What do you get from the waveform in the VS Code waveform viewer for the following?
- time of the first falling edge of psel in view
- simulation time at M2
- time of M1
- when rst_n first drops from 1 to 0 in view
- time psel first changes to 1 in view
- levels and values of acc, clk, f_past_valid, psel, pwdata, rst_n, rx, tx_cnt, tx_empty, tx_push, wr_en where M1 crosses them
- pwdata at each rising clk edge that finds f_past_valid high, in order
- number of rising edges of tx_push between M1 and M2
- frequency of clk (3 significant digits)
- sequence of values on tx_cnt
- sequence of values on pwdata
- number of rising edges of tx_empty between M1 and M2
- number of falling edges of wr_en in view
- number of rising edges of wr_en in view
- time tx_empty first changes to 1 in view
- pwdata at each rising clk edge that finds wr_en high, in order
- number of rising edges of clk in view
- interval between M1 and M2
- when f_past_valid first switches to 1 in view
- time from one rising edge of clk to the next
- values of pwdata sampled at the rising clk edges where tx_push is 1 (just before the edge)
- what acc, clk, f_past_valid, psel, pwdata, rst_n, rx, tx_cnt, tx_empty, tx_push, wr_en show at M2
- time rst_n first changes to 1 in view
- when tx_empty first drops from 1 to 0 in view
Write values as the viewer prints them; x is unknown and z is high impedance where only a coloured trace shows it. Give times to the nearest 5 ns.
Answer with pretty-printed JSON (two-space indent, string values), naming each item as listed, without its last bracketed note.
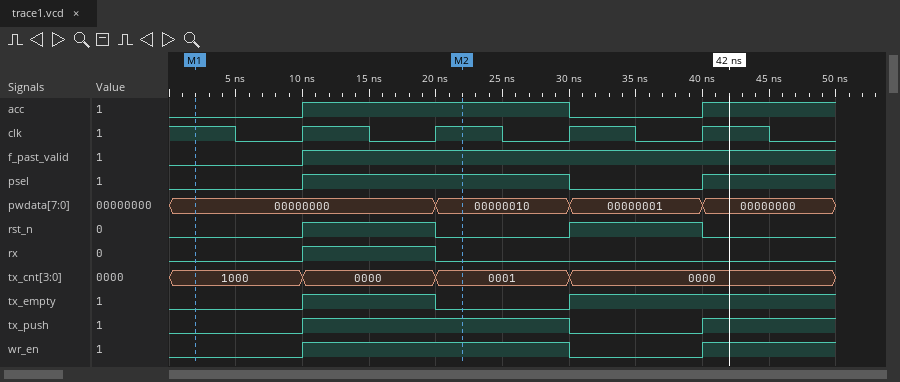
{
  "time of the first falling edge of psel in view": "30 ns",
  "simulation time at M2": "20 ns",
  "time of M1": "0 ns",
  "when rst_n first drops from 1 to 0 in view": "20 ns",
  "time psel first changes to 1 in view": "10 ns",
  "levels and values of acc, clk, f_past_valid, psel, pwdata, rst_n, rx, tx_cnt, tx_empty, tx_push, wr_en where M1 crosses them": "acc=0, clk=1, f_past_valid=0, psel=0, pwdata=00000000, rst_n=0, rx=0, tx_cnt=1000, tx_empty=0, tx_push=0, wr_en=0",
  "pwdata at each rising clk edge that finds f_past_valid high, in order": "00000000, 00000010, 00000001",
  "number of rising edges of tx_push between M1 and M2": "1",
  "frequency of clk": "100 MHz",
  "sequence of values on tx_cnt": "1000, 0000, 0001, 0000",
  "sequence of values on pwdata": "00000000, 00000010, 00000001, 00000000",
  "number of rising edges of tx_empty between M1 and M2": "1",
  "number of falling edges of wr_en in view": "1",
  "number of rising edges of wr_en in view": "2",
  "time tx_empty first changes to 1 in view": "10 ns",
  "pwdata at each rising clk edge that finds wr_en high, in order": "00000000, 00000010",
  "number of rising edges of clk in view": "4",
  "interval between M1 and M2": "20 ns",
  "when f_past_valid first switches to 1 in view": "10 ns",
  "time from one rising edge of clk to the next": "10 ns",
  "values of pwdata sampled at the rising clk edges where tx_push is 1": "00000000, 00000010",
  "what acc, clk, f_past_valid, psel, pwdata, rst_n, rx, tx_cnt, tx_empty, tx_push, wr_en show at M2": "acc=1, clk=1, f_past_valid=1, psel=1, pwdata=00000010, rst_n=0, rx=0, tx_cnt=0001, tx_empty=0, tx_push=1, wr_en=1",
  "time rst_n first changes to 1 in view": "10 ns",
  "when tx_empty first drops from 1 to 0 in view": "20 ns"
}
